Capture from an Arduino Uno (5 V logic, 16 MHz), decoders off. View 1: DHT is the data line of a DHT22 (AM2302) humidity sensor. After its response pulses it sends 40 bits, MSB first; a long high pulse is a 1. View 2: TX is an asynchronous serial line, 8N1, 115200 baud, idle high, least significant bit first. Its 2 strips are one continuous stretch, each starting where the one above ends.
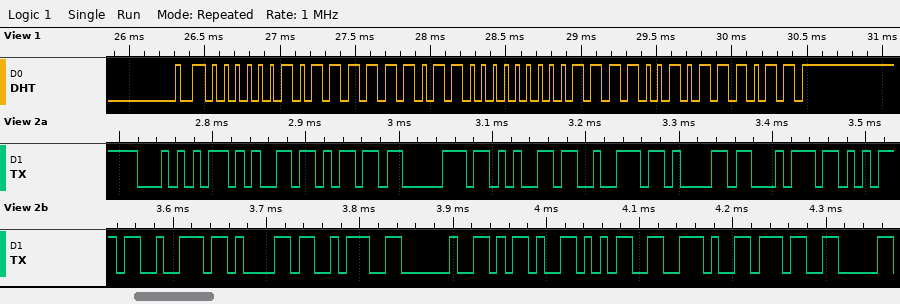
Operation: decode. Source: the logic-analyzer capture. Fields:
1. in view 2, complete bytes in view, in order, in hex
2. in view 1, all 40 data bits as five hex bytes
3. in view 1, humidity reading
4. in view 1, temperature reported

0x54 0x65 0x6D 0x70 0x65 0x72 0x61 0x74 0x75 0x72 0x61 0x3A 0x20 0x2D 0x35 0x2E 0x37
02 FD 80 3C BB
76.5 %
-6.0 °C
